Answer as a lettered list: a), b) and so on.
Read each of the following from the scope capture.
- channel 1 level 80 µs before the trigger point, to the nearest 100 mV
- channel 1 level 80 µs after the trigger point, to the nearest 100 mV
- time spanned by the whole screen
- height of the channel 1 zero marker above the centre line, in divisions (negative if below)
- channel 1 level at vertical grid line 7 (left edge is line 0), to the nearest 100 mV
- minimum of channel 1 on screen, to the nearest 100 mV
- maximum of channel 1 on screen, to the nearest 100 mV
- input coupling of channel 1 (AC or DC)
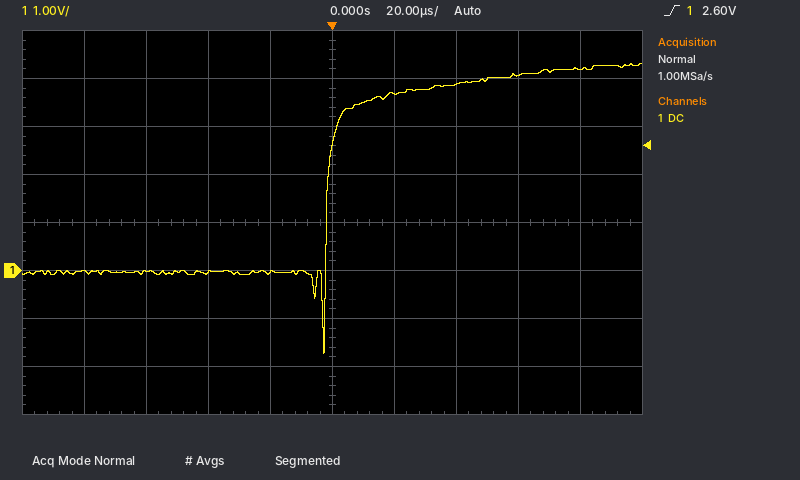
a) 0.0 V
b) 4.2 V
c) 200 µs
d) -1.0 div
e) 3.9 V
f) -1.7 V
g) 4.3 V
h) DC
